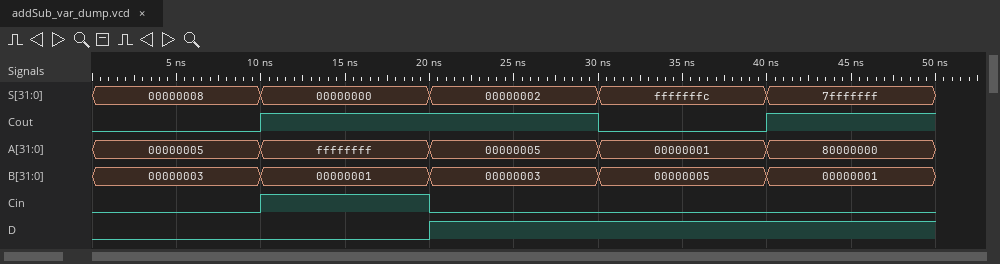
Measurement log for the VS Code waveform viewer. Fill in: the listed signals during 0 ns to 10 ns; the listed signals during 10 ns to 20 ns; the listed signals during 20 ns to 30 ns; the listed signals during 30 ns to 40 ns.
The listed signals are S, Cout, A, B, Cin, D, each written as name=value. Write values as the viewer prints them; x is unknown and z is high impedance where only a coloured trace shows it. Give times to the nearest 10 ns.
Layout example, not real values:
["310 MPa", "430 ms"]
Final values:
["S=00000008, Cout=0, A=00000005, B=00000003, Cin=0, D=0", "S=00000000, Cout=1, A=ffffffff, B=00000001, Cin=1, D=0", "S=00000002, Cout=1, A=00000005, B=00000003, Cin=0, D=1", "S=fffffffc, Cout=0, A=00000001, B=00000005, Cin=0, D=1"]
